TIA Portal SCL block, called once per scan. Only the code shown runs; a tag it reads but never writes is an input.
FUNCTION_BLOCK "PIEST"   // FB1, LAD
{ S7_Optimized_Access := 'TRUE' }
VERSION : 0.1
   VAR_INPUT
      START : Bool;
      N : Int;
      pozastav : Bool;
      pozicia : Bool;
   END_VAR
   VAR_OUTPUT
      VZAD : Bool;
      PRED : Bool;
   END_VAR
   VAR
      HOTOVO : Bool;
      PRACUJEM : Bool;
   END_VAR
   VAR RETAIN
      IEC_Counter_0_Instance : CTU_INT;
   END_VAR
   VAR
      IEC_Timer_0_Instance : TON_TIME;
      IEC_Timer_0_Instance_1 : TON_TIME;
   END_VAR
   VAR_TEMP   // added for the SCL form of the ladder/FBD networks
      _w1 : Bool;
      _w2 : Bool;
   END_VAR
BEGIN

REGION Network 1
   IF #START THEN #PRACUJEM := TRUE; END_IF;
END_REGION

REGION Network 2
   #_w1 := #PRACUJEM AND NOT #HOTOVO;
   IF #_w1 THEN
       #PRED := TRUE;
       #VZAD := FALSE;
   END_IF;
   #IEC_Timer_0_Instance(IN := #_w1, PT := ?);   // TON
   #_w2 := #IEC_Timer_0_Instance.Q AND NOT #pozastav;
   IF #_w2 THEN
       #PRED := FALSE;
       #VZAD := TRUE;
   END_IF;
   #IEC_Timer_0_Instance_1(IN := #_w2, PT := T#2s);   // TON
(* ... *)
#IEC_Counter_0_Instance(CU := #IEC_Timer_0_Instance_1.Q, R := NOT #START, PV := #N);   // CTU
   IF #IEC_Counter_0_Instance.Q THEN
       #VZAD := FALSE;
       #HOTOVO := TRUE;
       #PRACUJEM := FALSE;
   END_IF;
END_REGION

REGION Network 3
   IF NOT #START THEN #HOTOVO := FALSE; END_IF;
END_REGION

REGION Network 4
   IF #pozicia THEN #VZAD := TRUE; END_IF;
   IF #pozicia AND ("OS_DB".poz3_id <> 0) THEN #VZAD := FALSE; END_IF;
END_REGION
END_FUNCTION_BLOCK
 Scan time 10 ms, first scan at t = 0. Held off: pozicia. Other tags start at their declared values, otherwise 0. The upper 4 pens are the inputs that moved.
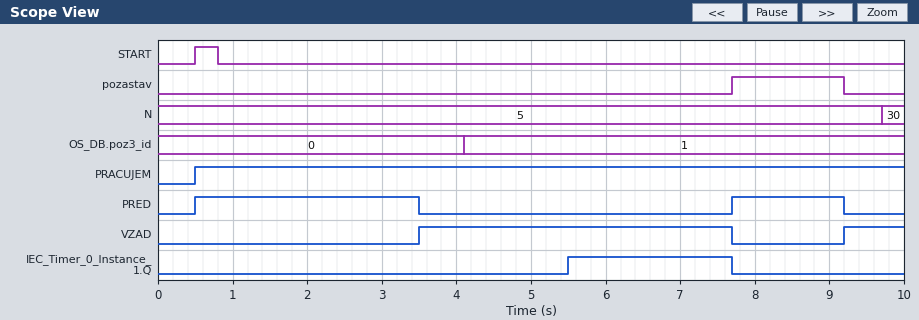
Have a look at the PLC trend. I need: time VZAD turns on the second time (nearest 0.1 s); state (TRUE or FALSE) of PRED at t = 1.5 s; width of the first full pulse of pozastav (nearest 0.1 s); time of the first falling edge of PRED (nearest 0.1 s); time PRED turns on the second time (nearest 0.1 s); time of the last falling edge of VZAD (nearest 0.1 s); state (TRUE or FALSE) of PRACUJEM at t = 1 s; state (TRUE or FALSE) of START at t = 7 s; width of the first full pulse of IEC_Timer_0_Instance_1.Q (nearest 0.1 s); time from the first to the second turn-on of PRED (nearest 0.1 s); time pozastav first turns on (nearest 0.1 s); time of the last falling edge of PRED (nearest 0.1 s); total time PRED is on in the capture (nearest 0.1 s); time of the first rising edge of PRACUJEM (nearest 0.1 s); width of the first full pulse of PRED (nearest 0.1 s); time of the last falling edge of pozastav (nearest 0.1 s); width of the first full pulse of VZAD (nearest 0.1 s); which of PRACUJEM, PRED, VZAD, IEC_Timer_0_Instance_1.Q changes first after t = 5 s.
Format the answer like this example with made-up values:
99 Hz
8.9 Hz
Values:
9.2 s
TRUE
1.5 s
3.5 s
7.7 s
7.7 s
TRUE
FALSE
2.2 s
7.2 s
7.7 s
9.2 s
4.5 s
0.5 s
3.0 s
9.2 s
4.2 s
IEC_Timer_0_Instance_1.Q
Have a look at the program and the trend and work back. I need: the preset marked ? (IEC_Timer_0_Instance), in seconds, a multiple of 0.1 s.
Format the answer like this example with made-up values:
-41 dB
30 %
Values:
3.0 s
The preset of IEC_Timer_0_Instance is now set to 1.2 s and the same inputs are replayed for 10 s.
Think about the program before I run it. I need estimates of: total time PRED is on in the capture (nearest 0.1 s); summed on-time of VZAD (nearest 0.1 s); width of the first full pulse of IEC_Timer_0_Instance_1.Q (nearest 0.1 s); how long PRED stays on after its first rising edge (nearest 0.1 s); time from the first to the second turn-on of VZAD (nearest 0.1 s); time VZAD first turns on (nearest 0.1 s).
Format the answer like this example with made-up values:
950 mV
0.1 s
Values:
2.7 s
6.8 s
4.0 s
1.2 s
7.5 s
1.7 s
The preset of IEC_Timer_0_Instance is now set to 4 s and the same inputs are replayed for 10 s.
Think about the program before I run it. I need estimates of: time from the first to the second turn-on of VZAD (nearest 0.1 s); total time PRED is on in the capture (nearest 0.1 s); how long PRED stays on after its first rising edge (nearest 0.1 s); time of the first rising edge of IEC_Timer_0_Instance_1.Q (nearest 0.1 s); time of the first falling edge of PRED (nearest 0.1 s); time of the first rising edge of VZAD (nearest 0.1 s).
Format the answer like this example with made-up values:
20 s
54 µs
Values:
4.7 s
5.5 s
4.0 s
6.5 s
4.5 s
4.5 s
